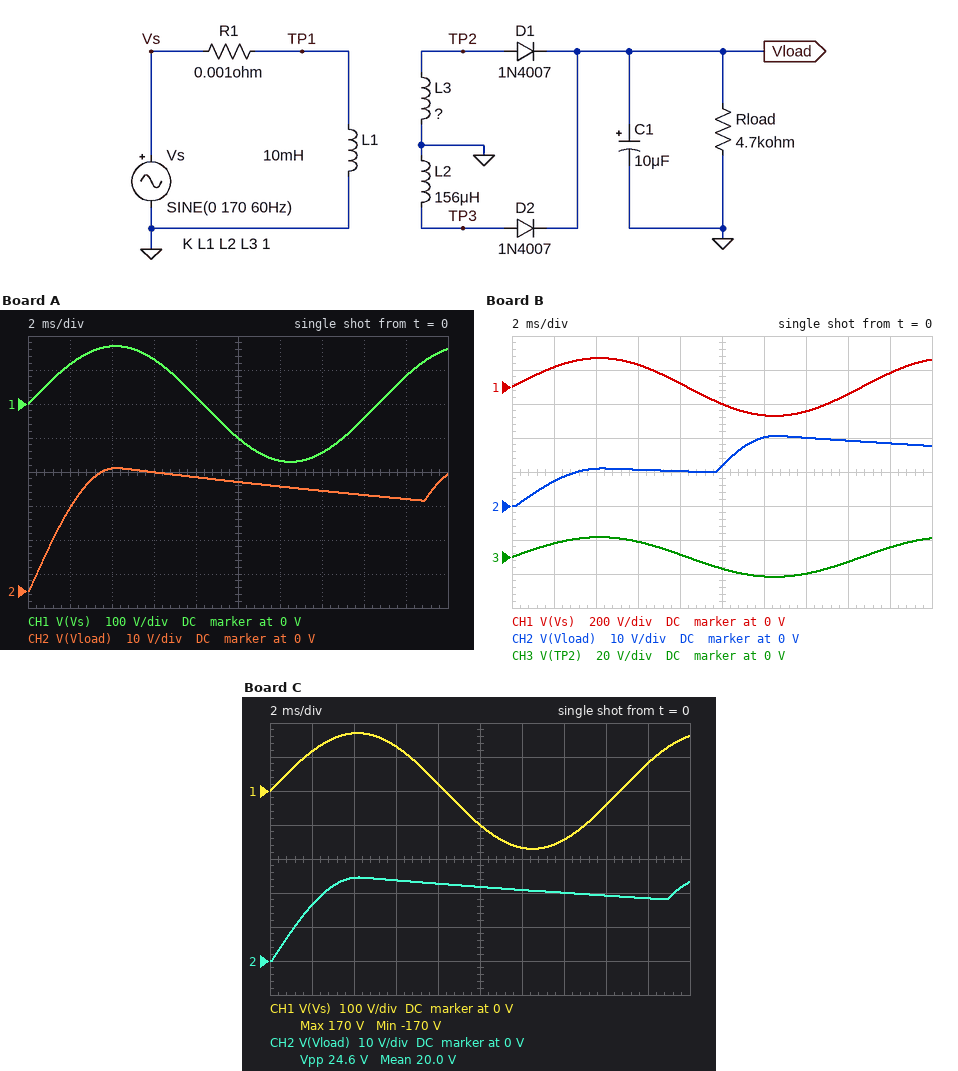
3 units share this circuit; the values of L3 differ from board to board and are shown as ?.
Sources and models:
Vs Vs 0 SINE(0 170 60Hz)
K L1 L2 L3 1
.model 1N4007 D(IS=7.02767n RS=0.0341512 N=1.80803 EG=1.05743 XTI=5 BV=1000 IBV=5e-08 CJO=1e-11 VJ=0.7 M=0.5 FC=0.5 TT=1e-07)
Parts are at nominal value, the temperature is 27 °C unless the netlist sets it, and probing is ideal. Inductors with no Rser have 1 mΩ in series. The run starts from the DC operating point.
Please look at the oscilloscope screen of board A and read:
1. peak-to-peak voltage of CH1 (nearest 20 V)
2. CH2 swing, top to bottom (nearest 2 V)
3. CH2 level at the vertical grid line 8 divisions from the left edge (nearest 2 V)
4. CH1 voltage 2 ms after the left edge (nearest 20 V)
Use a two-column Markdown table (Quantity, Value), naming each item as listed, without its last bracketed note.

| Quantity | Value |
|---|---|
| peak-to-peak voltage of CH1 | 340 V |
| CH2 swing, top to bottom | 36 V |
| CH2 level at the vertical grid line 8 divisions from the left edge | 28 V |
| CH1 voltage 2 ms after the left edge | 120 V |
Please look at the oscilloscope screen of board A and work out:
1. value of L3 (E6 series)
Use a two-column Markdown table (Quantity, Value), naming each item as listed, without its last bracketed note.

| Quantity | Value |
|---|---|
| value of L3 | 470 µH |
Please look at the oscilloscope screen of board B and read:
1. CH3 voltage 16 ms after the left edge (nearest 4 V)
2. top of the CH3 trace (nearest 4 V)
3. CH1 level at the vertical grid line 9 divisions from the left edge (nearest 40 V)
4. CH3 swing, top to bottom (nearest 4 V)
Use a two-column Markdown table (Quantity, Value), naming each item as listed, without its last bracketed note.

| Quantity | Value |
|---|---|
| CH3 voltage 16 ms after the left edge | -4 V |
| top of the CH3 trace | 12 V |
| CH1 level at the vertical grid line 9 divisions from the left edge | 80 V |
| CH3 swing, top to bottom | 24 V |
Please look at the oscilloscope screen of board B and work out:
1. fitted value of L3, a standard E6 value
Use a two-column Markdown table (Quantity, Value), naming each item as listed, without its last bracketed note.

| Quantity | Value |
|---|---|
| fitted value of L3, a standard E6 value | 47 µH |
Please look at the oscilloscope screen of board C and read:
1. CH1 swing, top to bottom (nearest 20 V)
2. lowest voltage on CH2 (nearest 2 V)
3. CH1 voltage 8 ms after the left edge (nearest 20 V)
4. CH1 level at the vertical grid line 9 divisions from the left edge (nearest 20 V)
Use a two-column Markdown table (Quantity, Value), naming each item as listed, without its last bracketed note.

| Quantity | Value |
|---|---|
| CH1 swing, top to bottom | 340 V |
| lowest voltage on CH2 | 0 V |
| CH1 voltage 8 ms after the left edge | 20 V |
| CH1 level at the vertical grid line 9 divisions from the left edge | 80 V |
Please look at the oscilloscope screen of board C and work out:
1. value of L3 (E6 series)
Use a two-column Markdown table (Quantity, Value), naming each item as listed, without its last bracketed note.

| Quantity | Value |
|---|---|
| value of L3 | 220 µH |
